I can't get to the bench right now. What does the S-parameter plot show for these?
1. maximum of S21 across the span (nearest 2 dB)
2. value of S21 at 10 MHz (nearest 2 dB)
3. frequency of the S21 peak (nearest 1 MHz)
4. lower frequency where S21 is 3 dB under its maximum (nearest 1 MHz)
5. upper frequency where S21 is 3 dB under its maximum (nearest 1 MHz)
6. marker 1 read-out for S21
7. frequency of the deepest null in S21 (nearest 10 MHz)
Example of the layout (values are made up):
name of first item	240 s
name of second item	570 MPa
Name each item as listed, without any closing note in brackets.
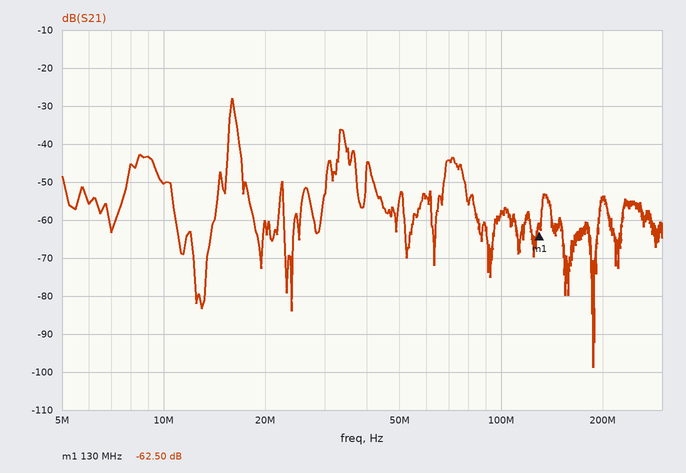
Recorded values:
maximum of S21 across the span	-28 dB
value of S21 at 10 MHz	-50 dB
frequency of the S21 peak	16 MHz
lower frequency where S21 is 3 dB under its maximum	16 MHz
upper frequency where S21 is 3 dB under its maximum	16 MHz
marker 1 read-out for S21	-62.50 dB
frequency of the deepest null in S21	190 MHz
